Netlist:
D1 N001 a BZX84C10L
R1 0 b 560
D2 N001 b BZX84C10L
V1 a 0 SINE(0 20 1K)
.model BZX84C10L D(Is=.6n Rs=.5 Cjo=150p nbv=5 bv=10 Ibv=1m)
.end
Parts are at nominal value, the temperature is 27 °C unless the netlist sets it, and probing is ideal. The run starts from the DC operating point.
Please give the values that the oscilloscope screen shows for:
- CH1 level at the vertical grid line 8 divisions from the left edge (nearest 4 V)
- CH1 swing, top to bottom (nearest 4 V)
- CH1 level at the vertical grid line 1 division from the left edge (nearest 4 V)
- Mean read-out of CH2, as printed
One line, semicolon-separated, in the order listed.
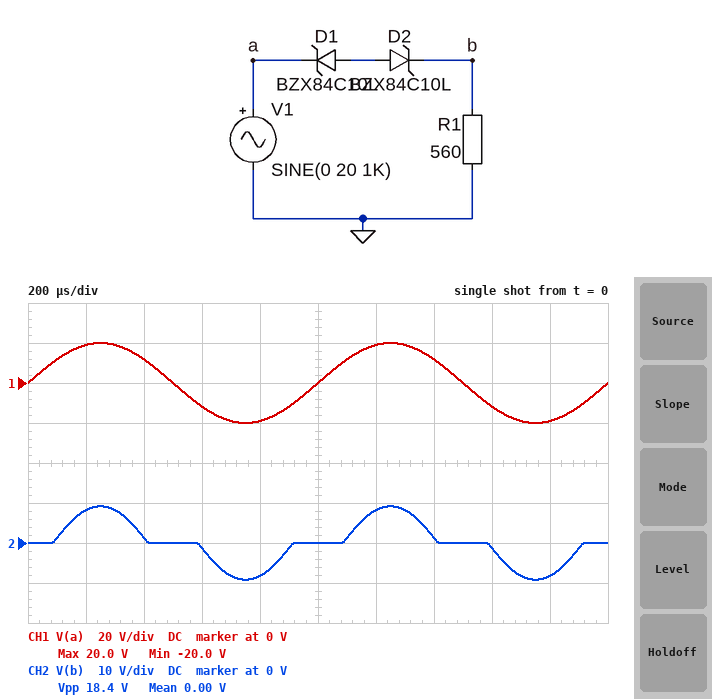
-12 V; 40 V; 20 V; 0.00 V
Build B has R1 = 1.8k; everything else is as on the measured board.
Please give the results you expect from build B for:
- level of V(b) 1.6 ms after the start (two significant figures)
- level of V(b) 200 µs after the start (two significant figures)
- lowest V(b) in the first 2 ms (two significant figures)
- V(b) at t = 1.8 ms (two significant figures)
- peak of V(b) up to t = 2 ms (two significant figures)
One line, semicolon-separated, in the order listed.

-1.4 V; 8.4 V; -9.4 V; -8.4 V; 9.4 V
